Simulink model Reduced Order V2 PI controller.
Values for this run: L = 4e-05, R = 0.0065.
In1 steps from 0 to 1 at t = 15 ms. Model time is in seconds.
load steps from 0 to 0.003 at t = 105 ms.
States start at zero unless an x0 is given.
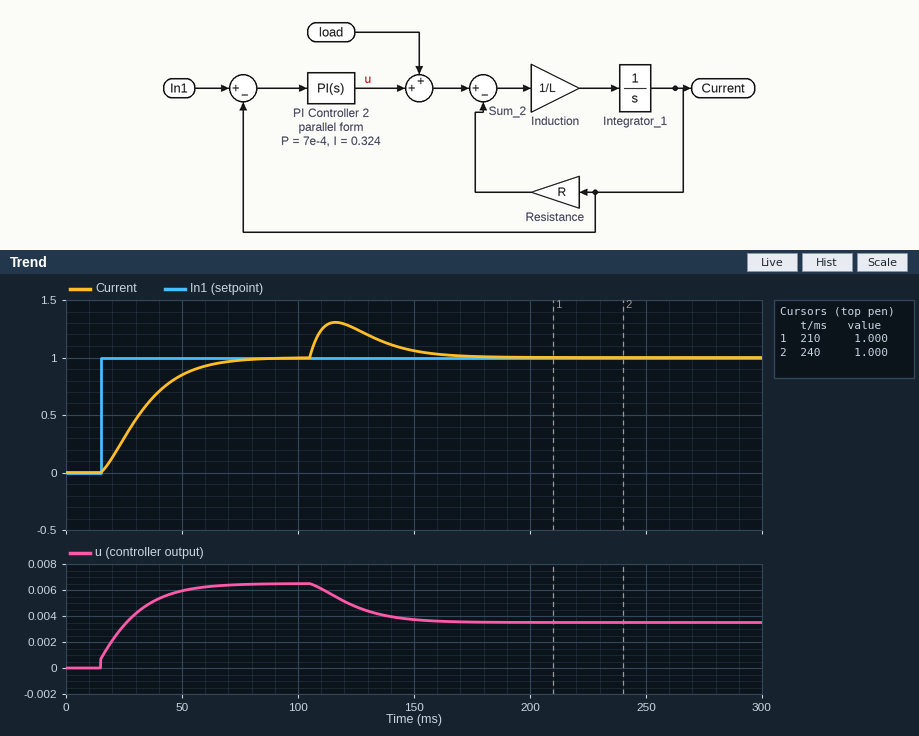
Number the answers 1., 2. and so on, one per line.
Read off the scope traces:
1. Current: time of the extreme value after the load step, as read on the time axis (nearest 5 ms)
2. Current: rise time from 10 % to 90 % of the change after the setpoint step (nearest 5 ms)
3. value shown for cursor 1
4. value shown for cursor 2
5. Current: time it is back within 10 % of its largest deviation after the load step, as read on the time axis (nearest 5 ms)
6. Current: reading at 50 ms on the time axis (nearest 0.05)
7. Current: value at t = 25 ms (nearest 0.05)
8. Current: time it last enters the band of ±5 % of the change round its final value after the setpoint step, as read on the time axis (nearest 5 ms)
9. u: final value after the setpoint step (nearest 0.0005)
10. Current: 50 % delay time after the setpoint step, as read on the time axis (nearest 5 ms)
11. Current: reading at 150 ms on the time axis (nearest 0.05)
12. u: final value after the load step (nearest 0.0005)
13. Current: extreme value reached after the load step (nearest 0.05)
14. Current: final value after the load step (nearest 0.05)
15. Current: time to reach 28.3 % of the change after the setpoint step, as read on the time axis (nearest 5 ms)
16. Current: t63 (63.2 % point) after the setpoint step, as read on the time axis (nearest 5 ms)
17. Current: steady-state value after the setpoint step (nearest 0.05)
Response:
1. 115 ms
2. 35 ms
3. 1.000
4. 1.000
5. 160 ms
6. 0.85
7. 0.30
8. 65 ms
9. 0.0065
10. 30 ms
11. 1.05
12. 0.0035
13. 1.30
14. 1.00
15. 25 ms
16. 35 ms
17. 1.00
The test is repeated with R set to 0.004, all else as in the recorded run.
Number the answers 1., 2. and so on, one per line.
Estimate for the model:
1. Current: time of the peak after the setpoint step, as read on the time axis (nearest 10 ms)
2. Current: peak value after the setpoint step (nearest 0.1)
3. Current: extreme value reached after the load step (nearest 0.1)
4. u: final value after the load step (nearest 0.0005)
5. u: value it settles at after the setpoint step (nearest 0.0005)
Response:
1. 60 ms
2. 1.1
3. 1.4
4. 0.0010
5. 0.0040
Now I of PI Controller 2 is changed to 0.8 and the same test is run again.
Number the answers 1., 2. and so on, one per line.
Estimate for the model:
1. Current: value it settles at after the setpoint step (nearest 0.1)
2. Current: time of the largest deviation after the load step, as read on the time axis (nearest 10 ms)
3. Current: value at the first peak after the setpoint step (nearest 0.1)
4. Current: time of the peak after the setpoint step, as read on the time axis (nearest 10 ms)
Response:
1. 1.0
2. 110 ms
3. 1.1
4. 40 ms
